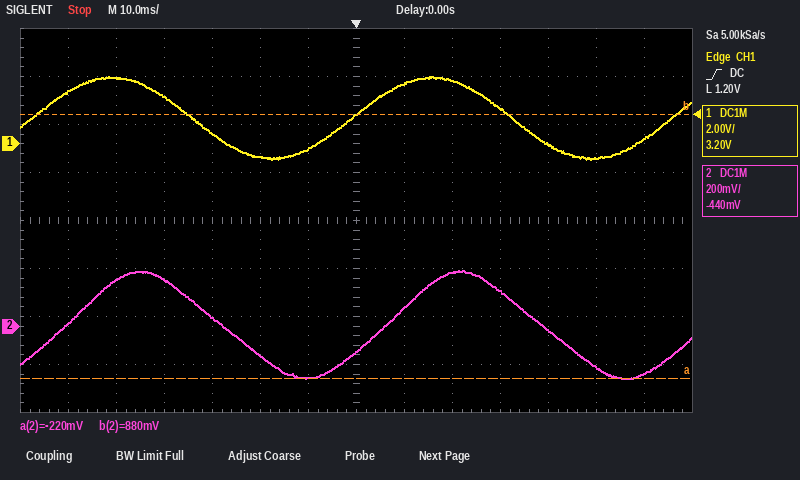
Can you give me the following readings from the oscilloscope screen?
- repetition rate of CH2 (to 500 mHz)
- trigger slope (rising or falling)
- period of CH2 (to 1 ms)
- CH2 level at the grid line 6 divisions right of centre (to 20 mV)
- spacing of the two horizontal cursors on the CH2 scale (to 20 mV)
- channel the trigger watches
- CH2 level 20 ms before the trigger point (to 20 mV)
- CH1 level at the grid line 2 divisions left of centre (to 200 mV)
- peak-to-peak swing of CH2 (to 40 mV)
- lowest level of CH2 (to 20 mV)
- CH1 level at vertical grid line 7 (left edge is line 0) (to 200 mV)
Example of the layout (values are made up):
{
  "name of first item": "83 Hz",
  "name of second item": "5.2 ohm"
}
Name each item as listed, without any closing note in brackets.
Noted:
{
  "repetition rate of CH2": "15.0 Hz",
  "trigger slope": "rising",
  "period of CH2": "67 ms",
  "CH2 level at the grid line 6 divisions right of centre": "-200 mV",
  "spacing of the two horizontal cursors on the CH2 scale": "1.10 V",
  "channel the trigger watches": "CH1",
  "CH2 level 20 ms before the trigger point": "-120 mV",
  "CH1 level at the grid line 2 divisions left of centre": "-600 mV",
  "peak-to-peak swing of CH2": "440 mV",
  "lowest level of CH2": "-220 mV",
  "CH1 level at vertical grid line 7 (left edge is line 0)": "1.2 V"
}
